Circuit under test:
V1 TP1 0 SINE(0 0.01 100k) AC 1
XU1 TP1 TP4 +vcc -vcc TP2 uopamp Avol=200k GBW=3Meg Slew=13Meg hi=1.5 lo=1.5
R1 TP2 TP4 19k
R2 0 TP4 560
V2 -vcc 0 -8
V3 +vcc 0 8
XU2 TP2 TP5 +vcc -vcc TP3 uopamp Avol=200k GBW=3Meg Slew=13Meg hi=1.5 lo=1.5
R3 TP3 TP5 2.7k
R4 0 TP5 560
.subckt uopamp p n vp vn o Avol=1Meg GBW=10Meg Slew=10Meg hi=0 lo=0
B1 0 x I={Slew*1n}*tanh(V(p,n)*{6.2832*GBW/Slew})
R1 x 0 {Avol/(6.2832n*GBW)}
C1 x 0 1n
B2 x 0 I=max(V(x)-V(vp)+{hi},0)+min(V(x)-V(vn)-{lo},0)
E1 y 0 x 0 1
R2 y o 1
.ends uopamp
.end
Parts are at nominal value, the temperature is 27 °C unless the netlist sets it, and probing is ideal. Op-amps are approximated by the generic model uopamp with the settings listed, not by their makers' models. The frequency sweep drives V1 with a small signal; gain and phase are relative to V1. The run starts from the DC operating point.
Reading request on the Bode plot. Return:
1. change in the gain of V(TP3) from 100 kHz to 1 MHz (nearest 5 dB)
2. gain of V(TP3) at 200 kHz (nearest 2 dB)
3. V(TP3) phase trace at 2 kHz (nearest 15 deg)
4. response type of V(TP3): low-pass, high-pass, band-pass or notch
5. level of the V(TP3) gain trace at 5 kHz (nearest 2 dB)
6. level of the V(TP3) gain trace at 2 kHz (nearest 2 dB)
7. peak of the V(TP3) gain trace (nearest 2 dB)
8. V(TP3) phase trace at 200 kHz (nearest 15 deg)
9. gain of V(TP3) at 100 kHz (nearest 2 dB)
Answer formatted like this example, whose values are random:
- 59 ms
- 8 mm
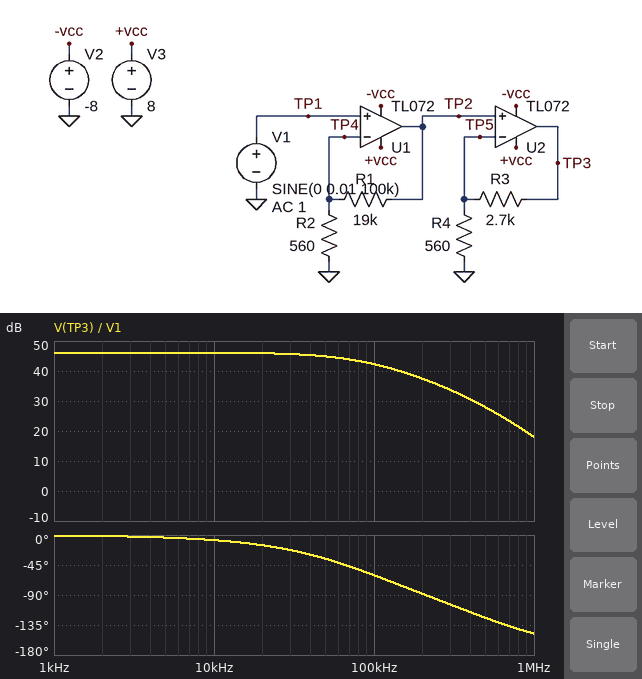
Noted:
- -25 dB
- 38 dB
- 0 deg
- low-pass
- 46 dB
- 46 dB
- 46 dB
- -90 deg
- 42 dB
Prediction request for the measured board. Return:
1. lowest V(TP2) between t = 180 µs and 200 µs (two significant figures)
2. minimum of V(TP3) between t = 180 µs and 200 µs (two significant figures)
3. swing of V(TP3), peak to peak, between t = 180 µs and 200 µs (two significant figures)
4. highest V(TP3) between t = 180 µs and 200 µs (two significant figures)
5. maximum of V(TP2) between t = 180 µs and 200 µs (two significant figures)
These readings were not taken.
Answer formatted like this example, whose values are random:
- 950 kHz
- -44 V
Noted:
- -230 mV
- -1.3 V
- 2.6 V
- 1.3 V
- 230 mV
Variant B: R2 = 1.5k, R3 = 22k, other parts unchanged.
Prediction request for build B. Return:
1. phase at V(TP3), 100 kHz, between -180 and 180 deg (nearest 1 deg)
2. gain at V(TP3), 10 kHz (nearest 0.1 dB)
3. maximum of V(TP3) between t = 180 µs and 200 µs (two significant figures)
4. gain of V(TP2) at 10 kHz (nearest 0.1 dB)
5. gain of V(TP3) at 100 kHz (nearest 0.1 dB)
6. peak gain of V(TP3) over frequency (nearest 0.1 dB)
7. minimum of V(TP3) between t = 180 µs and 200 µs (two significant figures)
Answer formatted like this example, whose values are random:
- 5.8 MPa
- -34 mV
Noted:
- -78 deg
- 54.7 dB
- 3.0 V
- 22.7 dB
- 49.5 dB
- 54.8 dB
- -3.0 V
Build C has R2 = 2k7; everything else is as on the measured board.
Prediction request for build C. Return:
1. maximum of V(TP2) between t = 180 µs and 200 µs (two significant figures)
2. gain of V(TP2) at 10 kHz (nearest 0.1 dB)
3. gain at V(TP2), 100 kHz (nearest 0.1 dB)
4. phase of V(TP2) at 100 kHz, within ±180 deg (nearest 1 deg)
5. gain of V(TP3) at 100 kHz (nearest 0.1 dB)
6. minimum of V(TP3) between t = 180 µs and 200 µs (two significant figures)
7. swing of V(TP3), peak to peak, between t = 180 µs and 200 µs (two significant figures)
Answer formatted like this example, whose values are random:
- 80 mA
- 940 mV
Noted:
- 78 mV
- 18.1 dB
- 17.8 dB
- -15 deg
- 32.9 dB
- -440 mV
- 890 mV
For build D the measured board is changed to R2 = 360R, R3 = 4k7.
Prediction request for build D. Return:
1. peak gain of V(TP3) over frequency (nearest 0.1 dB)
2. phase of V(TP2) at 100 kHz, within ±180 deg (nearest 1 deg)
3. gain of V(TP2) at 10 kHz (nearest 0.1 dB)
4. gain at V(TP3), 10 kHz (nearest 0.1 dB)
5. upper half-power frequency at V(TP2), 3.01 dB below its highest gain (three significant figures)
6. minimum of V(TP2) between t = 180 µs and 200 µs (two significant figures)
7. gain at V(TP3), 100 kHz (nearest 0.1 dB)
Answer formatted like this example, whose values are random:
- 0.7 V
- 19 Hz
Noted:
- 54.1 dB
- -61 deg
- 34.5 dB
- 53.9 dB
- 55.8 kHz
- -260 mV
- 47.4 dB
